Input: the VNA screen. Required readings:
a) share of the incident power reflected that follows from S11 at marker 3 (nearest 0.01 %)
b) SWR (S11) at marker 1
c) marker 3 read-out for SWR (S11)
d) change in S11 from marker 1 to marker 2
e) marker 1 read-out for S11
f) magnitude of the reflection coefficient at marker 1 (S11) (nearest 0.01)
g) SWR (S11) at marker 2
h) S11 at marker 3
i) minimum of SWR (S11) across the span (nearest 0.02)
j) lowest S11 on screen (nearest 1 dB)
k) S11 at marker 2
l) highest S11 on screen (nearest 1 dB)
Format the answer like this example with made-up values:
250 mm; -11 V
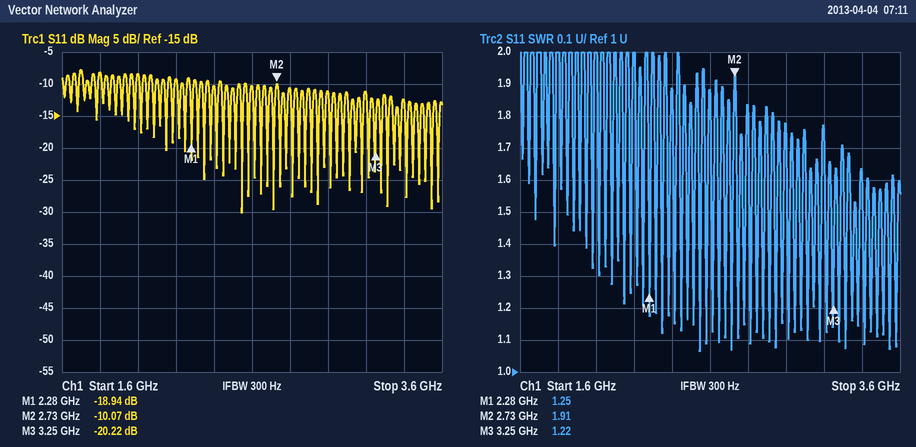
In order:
0.95 %; 1.25; 1.22; 8.87 dB; -18.94 dB; 0.11; 1.91; -20.22 dB; 1.06; -30 dB; -10.07 dB; -8 dB
